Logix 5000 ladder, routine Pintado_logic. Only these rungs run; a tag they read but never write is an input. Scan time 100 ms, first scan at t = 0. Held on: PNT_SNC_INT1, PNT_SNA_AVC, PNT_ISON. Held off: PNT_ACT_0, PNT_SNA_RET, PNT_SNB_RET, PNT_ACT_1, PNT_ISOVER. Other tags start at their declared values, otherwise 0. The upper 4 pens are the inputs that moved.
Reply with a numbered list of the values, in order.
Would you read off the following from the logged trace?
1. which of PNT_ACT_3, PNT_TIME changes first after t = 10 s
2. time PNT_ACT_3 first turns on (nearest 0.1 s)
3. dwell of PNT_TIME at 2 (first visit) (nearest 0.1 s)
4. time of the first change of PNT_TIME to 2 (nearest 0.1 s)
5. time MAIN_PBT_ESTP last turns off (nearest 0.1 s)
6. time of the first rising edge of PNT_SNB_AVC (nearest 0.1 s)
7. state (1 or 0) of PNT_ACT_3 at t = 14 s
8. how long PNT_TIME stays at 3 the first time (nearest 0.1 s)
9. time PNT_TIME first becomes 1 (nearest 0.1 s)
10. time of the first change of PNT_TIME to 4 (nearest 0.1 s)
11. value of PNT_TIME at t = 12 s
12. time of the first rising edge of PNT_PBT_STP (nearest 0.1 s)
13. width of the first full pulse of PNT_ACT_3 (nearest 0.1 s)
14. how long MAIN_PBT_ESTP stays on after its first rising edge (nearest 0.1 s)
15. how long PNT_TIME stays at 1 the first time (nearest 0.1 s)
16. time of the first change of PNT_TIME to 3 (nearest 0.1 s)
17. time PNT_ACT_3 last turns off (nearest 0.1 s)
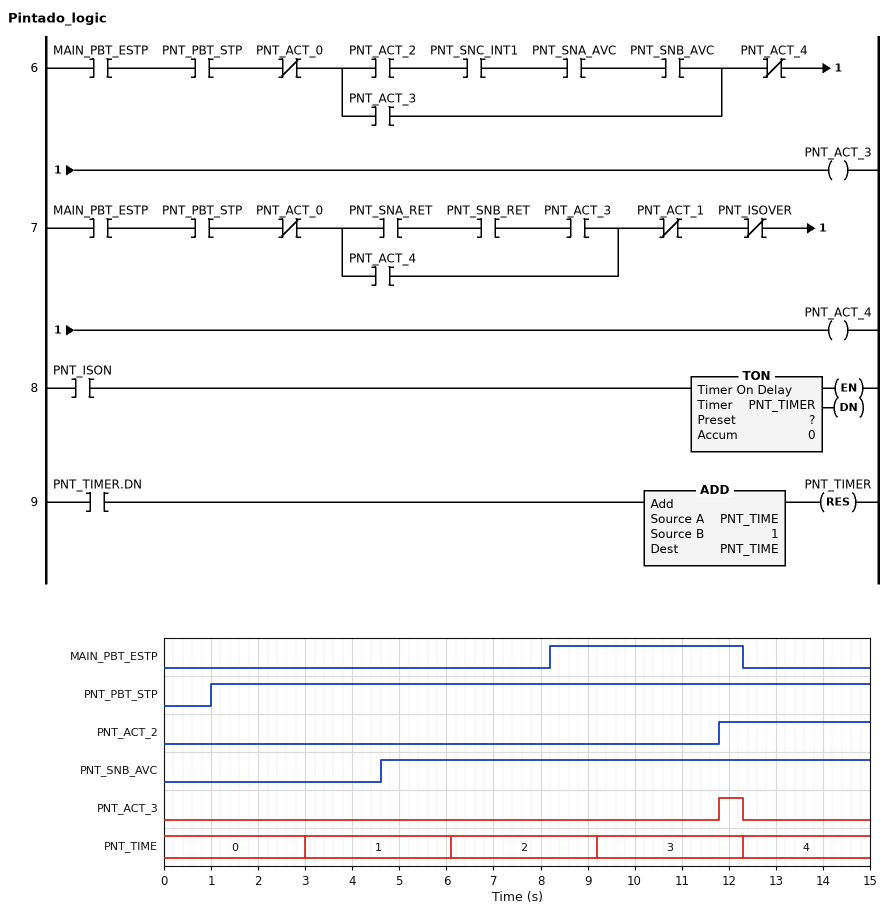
1. PNT_ACT_3
2. 11.8 s
3. 3.1 s
4. 6.1 s
5. 12.3 s
6. 4.6 s
7. 0
8. 3.1 s
9. 3.0 s
10. 12.3 s
11. 3
12. 1.0 s
13. 0.5 s
14. 4.1 s
15. 3.1 s
16. 9.2 s
17. 12.3 s
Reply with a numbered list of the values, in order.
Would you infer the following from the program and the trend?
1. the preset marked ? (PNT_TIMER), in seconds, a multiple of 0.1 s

1. 3.0 s
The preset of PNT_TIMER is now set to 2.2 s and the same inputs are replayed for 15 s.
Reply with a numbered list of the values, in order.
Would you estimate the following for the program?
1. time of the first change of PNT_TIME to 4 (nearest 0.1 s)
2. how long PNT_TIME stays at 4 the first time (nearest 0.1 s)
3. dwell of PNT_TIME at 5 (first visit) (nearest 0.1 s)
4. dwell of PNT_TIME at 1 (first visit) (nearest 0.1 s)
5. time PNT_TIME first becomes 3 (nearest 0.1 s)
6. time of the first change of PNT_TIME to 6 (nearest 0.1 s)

1. 9.1 s
2. 2.3 s
3. 2.3 s
4. 2.3 s
5. 6.8 s
6. 13.7 s
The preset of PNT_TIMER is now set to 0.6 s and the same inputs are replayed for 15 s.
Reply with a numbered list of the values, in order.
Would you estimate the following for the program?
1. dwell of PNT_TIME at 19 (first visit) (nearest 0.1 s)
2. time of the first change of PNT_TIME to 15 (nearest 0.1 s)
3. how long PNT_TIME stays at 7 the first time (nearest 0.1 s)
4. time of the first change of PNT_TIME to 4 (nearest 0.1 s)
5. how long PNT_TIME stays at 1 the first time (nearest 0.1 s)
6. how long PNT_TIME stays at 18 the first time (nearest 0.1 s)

1. 0.7 s
2. 10.4 s
3. 0.7 s
4. 2.7 s
5. 0.7 s
6. 0.7 s
